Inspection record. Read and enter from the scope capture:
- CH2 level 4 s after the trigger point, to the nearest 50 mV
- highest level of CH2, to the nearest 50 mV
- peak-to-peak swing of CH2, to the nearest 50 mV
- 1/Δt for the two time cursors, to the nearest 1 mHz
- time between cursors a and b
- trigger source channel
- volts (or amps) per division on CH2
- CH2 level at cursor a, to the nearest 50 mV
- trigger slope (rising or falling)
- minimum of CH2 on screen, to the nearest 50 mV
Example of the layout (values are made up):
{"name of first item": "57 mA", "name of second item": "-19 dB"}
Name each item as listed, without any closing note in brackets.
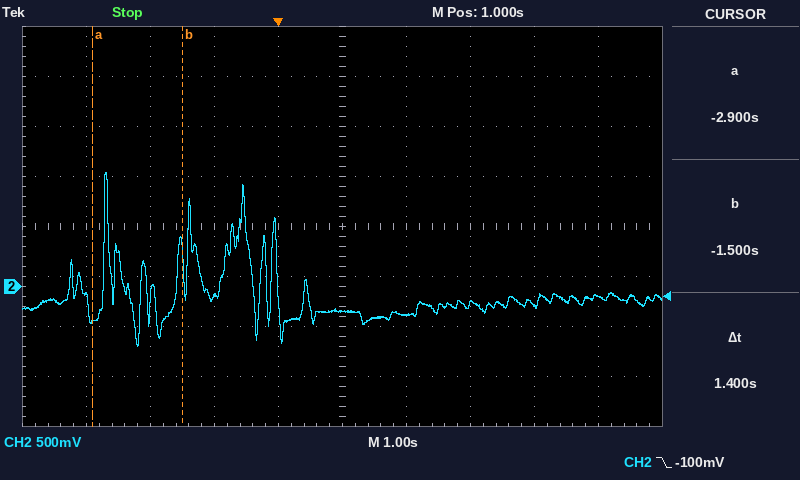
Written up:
{"CH2 level 4 s after the trigger point, to the nearest 50 mV": "-200 mV", "highest level of CH2, to the nearest 50 mV": "1.15 V", "peak-to-peak swing of CH2, to the nearest 50 mV": "1.75 V", "1/Δt for the two time cursors, to the nearest 1 mHz": "714 mHz", "time between cursors a and b": "1.4 s", "trigger source channel": "CH2", "volts (or amps) per division on CH2": "500 mV", "CH2 level at cursor a, to the nearest 50 mV": "-350 mV", "trigger slope": "falling", "minimum of CH2 on screen, to the nearest 50 mV": "-600 mV"}
